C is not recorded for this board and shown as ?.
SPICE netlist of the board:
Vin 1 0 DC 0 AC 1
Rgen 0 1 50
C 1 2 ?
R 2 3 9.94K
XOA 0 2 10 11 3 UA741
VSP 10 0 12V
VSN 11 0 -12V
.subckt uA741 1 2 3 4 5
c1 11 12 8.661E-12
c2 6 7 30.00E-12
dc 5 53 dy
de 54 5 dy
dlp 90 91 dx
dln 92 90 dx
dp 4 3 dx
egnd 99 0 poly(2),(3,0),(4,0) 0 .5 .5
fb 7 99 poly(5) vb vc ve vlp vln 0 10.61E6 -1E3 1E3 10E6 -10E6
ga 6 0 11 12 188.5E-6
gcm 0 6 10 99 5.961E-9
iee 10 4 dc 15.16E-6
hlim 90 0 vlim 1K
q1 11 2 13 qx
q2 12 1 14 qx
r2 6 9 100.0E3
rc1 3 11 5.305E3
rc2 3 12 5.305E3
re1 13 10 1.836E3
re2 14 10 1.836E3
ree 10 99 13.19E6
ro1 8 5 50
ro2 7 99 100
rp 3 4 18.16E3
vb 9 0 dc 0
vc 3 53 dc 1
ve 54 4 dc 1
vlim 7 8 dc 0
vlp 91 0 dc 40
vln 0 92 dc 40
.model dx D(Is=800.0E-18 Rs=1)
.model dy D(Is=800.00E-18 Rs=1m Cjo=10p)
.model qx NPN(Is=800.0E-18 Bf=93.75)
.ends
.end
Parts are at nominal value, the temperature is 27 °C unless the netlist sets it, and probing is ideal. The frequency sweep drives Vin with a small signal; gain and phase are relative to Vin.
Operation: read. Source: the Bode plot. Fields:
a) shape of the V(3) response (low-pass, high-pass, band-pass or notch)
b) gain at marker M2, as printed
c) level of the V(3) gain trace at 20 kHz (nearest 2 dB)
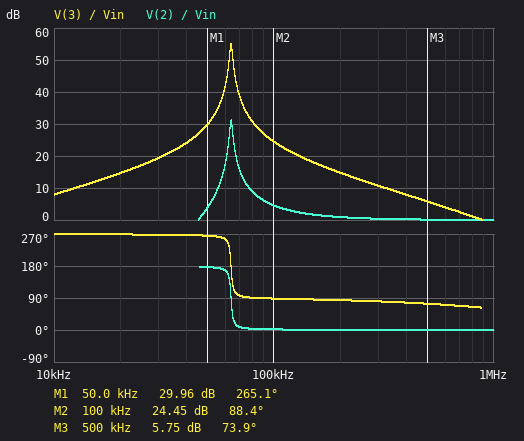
band-pass
24.45 dB
14 dB
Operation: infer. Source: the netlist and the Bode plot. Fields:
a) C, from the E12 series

3.9 nF
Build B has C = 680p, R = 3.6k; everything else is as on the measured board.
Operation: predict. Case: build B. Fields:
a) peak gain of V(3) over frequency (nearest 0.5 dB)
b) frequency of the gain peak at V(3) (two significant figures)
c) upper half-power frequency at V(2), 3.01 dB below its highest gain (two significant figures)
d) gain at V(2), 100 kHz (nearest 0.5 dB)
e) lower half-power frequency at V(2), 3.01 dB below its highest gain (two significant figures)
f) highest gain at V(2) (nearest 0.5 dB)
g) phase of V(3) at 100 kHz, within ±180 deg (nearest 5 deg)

31.0 dB
250 kHz
270 kHz
-14.5 dB
240 kHz
19.0 dB
-95 deg
